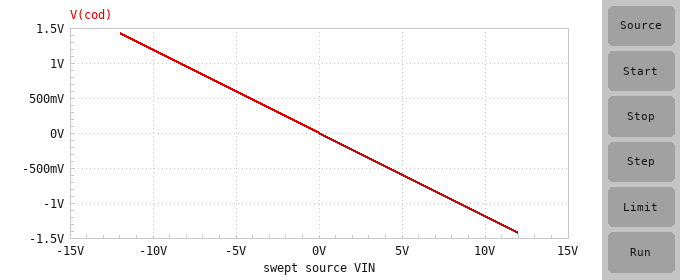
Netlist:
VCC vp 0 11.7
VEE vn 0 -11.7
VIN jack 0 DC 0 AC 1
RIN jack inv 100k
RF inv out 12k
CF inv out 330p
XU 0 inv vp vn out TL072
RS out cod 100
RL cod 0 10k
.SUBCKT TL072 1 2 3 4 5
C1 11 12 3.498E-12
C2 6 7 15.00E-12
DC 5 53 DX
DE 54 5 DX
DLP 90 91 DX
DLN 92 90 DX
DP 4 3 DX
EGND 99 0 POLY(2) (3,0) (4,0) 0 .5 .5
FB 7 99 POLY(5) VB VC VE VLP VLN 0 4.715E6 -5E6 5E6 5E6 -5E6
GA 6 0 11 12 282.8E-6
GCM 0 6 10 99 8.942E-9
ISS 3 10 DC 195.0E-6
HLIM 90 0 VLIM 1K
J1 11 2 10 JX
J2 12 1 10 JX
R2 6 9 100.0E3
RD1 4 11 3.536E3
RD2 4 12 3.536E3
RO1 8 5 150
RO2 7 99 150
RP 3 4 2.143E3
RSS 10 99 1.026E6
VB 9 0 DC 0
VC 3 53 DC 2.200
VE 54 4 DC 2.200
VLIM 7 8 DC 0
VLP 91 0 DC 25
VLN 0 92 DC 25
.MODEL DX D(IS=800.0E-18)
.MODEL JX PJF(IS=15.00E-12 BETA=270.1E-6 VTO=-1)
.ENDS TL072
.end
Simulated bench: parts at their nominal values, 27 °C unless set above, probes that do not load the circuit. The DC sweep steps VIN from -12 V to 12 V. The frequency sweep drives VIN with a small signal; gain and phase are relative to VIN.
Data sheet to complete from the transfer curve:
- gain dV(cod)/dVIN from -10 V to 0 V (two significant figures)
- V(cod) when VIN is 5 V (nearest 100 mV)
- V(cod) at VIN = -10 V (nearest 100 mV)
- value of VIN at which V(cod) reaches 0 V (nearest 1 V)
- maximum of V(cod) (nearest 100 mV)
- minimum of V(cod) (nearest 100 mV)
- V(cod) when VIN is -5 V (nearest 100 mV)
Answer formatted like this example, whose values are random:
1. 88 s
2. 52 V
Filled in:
1. -0.12 V/V
2. -600 mV
3. 1.2 V
4. 0 V
5. 1.4 V
6. -1.4 V
7. 600 mV
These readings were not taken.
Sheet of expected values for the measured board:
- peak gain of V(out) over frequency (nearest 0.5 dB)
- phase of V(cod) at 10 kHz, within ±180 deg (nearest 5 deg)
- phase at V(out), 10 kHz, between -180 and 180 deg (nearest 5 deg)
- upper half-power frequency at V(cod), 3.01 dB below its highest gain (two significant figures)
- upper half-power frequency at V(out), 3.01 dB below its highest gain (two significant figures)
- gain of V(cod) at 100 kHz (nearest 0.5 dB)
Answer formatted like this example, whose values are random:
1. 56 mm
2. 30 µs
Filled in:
1. -18.5 dB
2. 165 deg
3. 165 deg
4. 40 kHz
5. 40 kHz
6. -27.0 dB
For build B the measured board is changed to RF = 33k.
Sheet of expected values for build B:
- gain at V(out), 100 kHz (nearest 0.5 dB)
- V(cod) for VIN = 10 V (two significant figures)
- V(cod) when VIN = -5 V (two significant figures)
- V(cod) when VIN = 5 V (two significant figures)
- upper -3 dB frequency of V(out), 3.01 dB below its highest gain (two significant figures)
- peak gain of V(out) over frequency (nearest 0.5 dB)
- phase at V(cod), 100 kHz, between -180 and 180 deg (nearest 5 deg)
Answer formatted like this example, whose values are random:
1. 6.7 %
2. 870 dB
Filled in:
1. -26.5 dB
2. -3.3 V
3. 1.6 V
4. -1.6 V
5. 15 kHz
6. -9.5 dB
7. 95 deg
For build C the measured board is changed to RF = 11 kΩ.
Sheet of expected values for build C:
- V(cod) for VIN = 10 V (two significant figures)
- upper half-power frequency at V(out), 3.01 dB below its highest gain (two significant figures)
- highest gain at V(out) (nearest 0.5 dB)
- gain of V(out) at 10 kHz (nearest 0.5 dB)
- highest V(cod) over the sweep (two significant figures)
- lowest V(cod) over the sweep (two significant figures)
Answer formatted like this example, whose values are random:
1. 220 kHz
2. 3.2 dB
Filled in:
1. -1.1 V
2. 44 kHz
3. -19.0 dB
4. -19.5 dB
5. 1.3 V
6. -1.3 V
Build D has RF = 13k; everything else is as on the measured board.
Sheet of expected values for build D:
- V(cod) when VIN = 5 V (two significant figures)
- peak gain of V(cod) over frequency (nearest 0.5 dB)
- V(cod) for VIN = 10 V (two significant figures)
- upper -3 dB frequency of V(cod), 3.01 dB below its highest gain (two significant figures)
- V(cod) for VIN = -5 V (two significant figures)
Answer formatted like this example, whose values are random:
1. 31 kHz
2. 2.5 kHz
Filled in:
1. -640 mV
2. -18.0 dB
3. -1.3 V
4. 37 kHz
5. 640 mV
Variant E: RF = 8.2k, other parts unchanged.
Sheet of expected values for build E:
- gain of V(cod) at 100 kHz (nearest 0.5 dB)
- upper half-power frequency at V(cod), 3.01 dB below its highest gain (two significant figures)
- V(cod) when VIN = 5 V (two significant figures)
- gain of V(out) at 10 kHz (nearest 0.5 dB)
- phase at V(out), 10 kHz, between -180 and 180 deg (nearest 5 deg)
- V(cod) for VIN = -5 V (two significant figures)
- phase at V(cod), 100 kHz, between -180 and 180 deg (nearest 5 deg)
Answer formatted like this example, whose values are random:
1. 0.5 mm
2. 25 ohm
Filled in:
1. -27.5 dB
2. 59 kHz
3. -410 mV
4. -22.0 dB
5. 170 deg
6. 410 mV
7. 120 deg
